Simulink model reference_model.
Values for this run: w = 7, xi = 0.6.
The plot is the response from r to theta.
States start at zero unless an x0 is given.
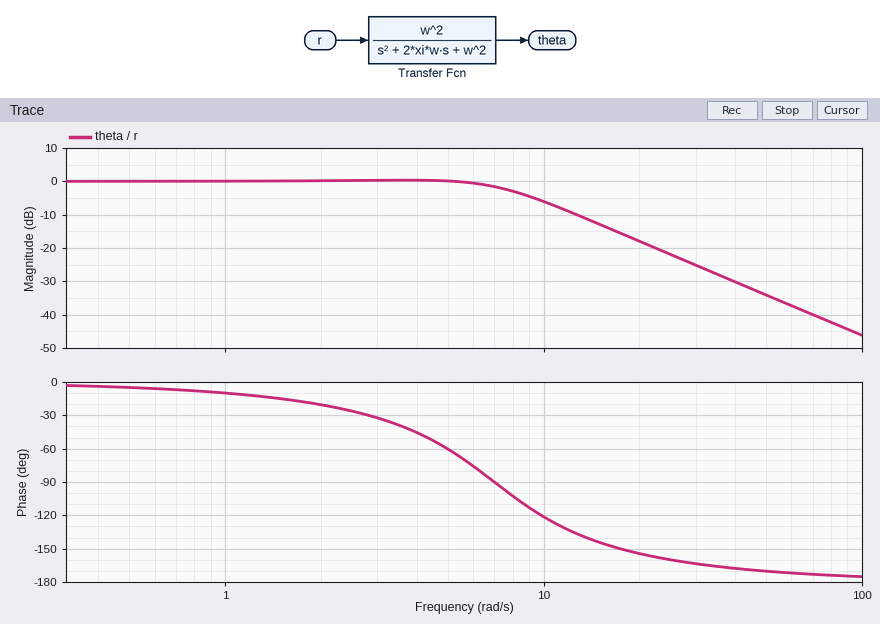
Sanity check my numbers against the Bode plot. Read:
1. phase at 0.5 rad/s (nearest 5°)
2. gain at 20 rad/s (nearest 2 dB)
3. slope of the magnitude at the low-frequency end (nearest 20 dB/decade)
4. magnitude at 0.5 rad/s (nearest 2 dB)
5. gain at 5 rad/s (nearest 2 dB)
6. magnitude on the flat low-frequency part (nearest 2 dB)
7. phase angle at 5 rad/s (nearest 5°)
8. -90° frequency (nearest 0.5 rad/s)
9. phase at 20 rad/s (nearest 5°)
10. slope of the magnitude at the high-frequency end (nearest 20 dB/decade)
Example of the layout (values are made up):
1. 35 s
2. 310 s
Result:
1. -5°
2. -18 dB
3. 0 dB/decade
4. 0 dB
5. 0 dB
6. 0 dB
7. -60°
8. 7.0 rad/s
9. -155°
10. -40 dB/decade
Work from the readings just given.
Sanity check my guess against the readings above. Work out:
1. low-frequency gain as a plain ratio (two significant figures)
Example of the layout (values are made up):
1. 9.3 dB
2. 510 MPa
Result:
1. 1.0
